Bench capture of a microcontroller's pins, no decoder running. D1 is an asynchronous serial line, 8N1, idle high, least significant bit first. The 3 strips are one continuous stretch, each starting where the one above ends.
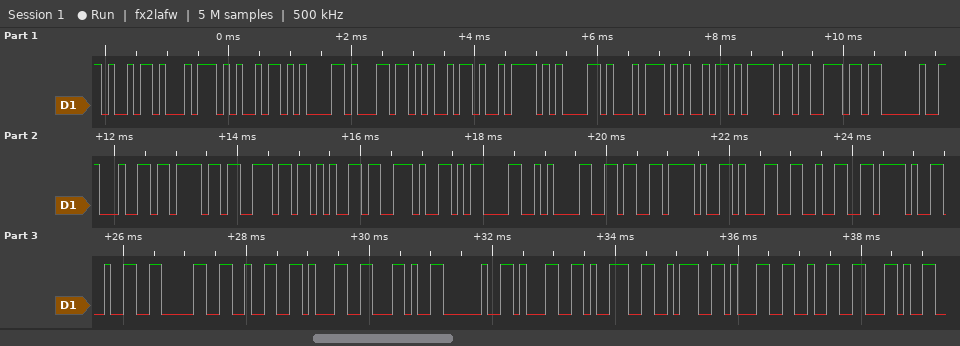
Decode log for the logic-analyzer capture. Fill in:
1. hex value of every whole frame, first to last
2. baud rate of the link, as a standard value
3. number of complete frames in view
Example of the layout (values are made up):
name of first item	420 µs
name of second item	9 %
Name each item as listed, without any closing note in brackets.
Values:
hex value of every whole frame, first to last	69 74 69 61 6C 69 7A 61 74 69 6F 6E 20 64 6F 6E 65 2E 0D 0A 36 2F 31 32 2F 32 30 32 31 2C 20 31 39 3A 31 32 2C
baud rate of the link, as a standard value	9600 baud
number of complete frames in view	37
